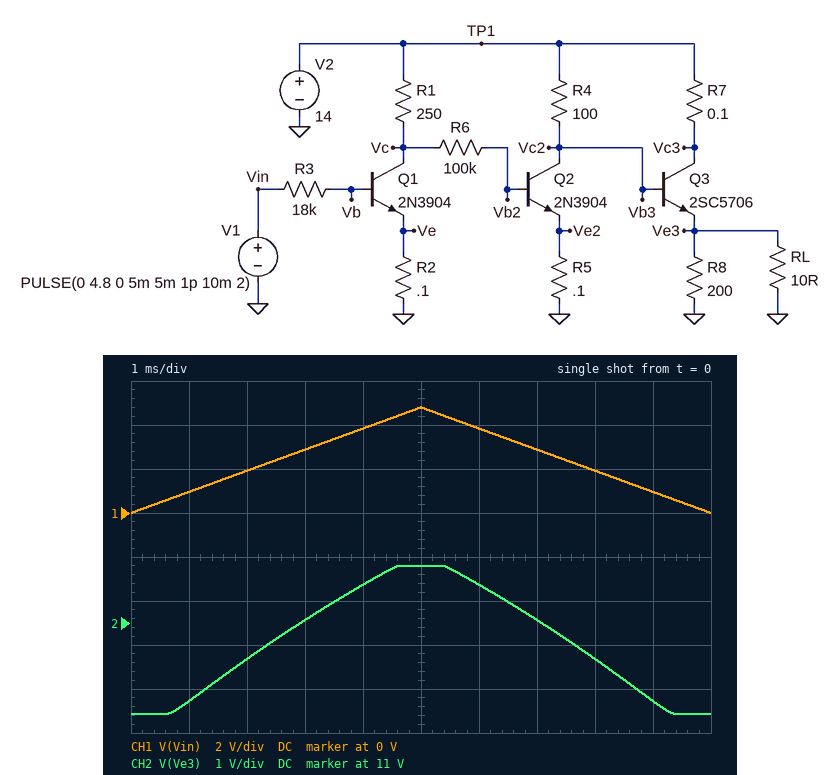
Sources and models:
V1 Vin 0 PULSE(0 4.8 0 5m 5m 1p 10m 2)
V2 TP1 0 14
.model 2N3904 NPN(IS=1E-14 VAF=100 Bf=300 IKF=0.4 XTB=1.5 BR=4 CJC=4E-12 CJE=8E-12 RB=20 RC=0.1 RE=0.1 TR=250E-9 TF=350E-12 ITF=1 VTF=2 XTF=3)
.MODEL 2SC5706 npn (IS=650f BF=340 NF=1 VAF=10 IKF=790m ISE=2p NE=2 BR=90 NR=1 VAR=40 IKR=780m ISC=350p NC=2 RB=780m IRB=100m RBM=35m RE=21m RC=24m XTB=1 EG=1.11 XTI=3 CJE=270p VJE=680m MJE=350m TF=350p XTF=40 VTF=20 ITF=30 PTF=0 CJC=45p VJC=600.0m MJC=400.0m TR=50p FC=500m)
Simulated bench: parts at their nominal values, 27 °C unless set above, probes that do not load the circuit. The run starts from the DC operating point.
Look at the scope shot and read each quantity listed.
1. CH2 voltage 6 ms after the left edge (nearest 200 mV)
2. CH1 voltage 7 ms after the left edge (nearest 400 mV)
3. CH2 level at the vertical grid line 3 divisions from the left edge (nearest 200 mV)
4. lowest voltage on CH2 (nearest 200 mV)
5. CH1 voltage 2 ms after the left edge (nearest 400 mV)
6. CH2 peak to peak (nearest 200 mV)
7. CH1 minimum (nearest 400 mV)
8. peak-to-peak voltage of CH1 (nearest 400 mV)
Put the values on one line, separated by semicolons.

11.8 V; 2.8 V; 11.0 V; 9.0 V; 2.0 V; 3.4 V; 0 V; 4.8 V
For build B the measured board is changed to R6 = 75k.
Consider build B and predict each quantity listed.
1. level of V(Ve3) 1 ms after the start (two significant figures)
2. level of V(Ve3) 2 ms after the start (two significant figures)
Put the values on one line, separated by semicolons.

8.3 V; 9.5 V
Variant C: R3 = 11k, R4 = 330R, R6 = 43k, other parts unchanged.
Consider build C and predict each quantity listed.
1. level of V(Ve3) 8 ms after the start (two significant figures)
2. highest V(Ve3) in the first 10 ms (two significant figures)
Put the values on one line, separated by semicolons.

1.6 V; 11 V
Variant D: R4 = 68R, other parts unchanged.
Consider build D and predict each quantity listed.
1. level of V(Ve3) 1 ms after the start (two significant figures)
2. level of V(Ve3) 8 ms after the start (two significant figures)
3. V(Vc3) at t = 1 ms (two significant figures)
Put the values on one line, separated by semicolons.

10 V; 11 V; 14 V
